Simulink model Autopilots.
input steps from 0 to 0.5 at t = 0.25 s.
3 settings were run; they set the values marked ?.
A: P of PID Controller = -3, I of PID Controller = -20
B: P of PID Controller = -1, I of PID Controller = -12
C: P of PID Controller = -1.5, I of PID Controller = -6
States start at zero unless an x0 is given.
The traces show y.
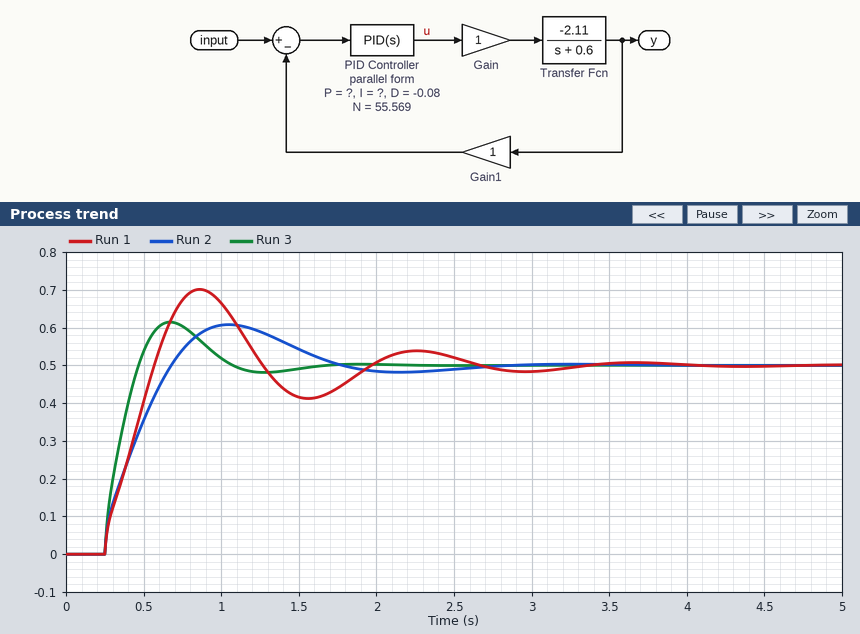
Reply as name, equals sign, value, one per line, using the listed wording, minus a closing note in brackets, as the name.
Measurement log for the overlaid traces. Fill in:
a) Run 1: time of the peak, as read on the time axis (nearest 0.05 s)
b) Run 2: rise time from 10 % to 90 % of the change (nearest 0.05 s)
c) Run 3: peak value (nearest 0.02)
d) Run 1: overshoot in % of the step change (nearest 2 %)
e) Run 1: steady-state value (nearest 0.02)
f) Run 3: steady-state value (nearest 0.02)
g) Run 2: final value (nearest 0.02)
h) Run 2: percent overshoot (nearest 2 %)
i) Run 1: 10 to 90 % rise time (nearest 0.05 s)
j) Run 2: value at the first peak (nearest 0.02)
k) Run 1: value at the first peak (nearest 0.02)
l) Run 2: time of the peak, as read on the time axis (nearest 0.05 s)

Run 1: time of the peak, as read on the time axis = 0.85 s
Run 2: rise time from 10 % to 90 % of the change = 0.35 s
Run 3: peak value = 0.62
Run 1: overshoot in % of the step change = 40 %
Run 1: steady-state value = 0.50
Run 3: steady-state value = 0.50
Run 2: final value = 0.50
Run 2: percent overshoot = 22 %
Run 1: 10 to 90 % rise time = 0.25 s
Run 2: value at the first peak = 0.60
Run 1: value at the first peak = 0.70
Run 2: time of the peak, as read on the time axis = 1.05 s
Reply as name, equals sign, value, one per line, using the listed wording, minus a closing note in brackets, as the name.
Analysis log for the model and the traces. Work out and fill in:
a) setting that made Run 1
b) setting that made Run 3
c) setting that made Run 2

setting that made Run 1 = B
setting that made Run 3 = A
setting that made Run 2 = C
